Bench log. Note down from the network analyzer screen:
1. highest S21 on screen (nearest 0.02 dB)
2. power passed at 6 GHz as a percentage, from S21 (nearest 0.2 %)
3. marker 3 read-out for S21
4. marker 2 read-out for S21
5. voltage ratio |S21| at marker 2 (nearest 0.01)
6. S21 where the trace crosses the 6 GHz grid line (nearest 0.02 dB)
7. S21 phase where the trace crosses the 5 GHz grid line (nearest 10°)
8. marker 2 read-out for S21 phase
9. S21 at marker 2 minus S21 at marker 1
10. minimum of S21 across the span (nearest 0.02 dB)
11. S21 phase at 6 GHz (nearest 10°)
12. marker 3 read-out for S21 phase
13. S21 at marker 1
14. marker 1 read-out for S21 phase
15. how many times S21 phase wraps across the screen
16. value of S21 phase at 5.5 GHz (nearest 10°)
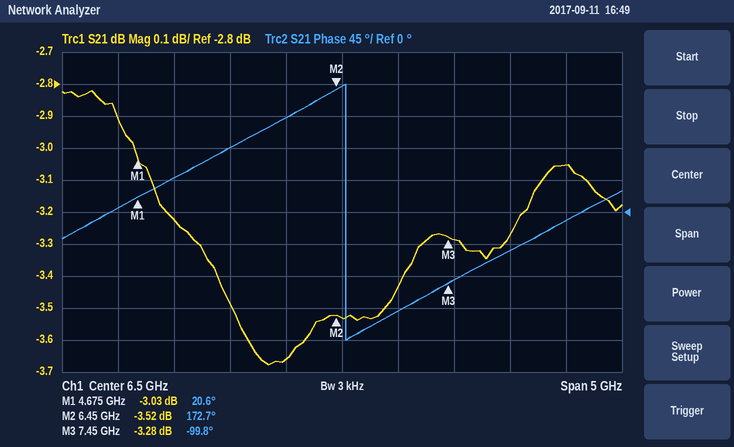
-2.82 dB
43.0 %
-3.28 dB
-3.52 dB
0.67
-3.66 dB
50°
172.7°
-0.49 dB
-3.68 dB
130°
-99.8°
-3.03 dB
20.6°
1
90°
